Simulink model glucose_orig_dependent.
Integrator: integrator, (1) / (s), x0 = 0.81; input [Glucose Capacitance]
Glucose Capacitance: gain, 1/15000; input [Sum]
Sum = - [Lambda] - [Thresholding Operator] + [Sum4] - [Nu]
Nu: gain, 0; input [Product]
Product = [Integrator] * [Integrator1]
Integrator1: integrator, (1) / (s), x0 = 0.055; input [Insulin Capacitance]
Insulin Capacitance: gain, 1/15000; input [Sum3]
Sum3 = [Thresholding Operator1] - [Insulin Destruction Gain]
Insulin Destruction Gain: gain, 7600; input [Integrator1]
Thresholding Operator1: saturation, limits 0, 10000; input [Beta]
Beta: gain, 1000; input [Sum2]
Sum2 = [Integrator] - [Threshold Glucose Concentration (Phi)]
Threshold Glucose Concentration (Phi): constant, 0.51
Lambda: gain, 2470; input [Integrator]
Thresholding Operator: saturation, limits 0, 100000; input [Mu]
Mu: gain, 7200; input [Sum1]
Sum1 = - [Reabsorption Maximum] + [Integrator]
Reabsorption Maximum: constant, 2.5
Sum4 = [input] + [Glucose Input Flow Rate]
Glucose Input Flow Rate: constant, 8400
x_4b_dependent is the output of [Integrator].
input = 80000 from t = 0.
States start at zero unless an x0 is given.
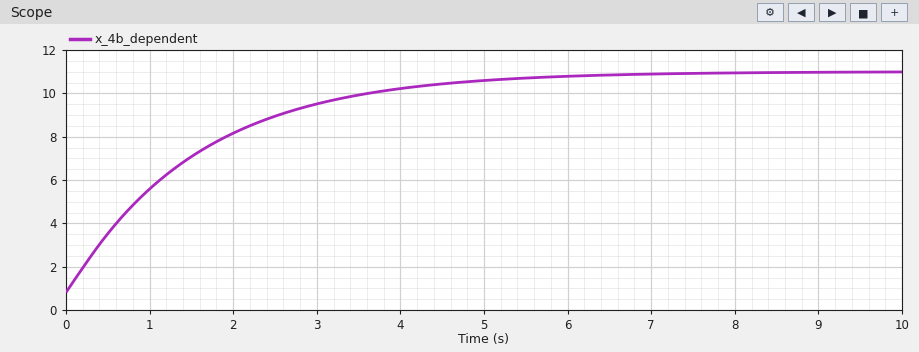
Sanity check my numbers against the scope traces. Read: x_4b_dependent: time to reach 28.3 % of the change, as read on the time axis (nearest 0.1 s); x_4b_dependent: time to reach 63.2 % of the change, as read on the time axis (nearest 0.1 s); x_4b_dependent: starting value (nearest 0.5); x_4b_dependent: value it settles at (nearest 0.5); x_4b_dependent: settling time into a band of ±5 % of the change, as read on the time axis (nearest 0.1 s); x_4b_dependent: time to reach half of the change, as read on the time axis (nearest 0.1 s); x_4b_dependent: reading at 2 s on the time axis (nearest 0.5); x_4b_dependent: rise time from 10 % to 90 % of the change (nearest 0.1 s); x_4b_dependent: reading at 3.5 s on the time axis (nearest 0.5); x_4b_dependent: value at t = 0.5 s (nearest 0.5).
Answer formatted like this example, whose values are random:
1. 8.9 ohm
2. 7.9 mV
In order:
1. 0.5 s
2. 1.6 s
3. 1.0
4. 11.0
5. 4.7 s
6. 1.1 s
7. 8.0
8. 3.4 s
9. 10.0
10. 3.5
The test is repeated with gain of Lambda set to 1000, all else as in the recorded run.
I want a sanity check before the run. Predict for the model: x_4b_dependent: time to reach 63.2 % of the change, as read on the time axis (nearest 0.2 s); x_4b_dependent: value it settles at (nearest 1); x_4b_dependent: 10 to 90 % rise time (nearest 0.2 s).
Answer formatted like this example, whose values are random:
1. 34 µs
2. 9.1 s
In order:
1. 1.8 s
2. 13
3. 4.0 s
